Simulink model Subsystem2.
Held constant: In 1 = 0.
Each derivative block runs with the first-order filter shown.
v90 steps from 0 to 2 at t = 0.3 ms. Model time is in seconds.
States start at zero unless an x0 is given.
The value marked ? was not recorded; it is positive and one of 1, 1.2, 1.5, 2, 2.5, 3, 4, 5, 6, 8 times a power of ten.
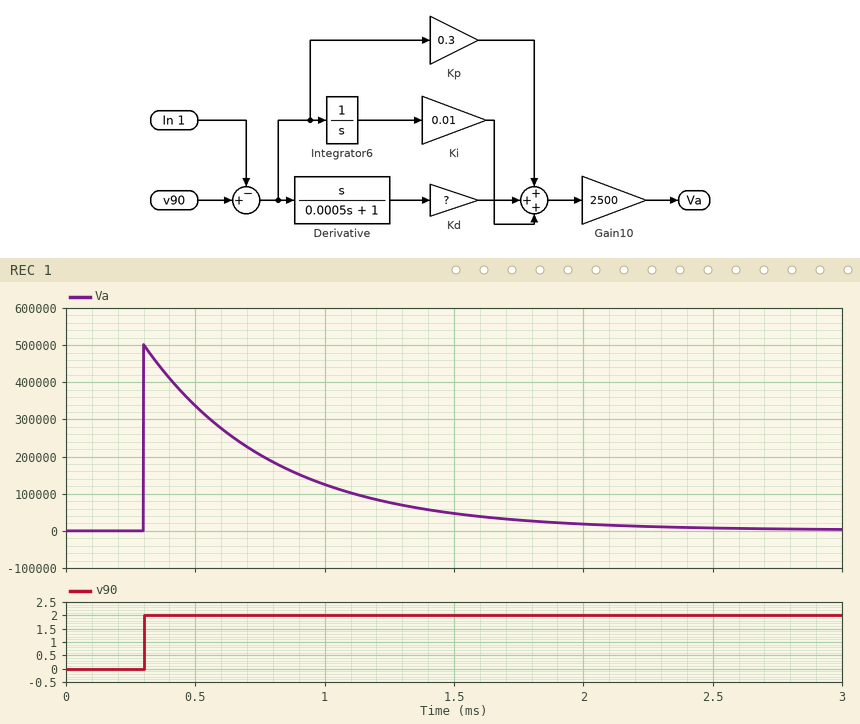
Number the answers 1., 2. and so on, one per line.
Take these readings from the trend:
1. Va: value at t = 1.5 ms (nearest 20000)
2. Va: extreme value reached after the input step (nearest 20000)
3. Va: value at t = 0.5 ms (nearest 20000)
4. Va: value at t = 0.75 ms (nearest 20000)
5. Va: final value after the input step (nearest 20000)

1. 40000
2. 500000
3. 340000
4. 200000
5. 0
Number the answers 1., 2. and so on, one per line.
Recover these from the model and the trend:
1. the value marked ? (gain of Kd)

1. 0.05
